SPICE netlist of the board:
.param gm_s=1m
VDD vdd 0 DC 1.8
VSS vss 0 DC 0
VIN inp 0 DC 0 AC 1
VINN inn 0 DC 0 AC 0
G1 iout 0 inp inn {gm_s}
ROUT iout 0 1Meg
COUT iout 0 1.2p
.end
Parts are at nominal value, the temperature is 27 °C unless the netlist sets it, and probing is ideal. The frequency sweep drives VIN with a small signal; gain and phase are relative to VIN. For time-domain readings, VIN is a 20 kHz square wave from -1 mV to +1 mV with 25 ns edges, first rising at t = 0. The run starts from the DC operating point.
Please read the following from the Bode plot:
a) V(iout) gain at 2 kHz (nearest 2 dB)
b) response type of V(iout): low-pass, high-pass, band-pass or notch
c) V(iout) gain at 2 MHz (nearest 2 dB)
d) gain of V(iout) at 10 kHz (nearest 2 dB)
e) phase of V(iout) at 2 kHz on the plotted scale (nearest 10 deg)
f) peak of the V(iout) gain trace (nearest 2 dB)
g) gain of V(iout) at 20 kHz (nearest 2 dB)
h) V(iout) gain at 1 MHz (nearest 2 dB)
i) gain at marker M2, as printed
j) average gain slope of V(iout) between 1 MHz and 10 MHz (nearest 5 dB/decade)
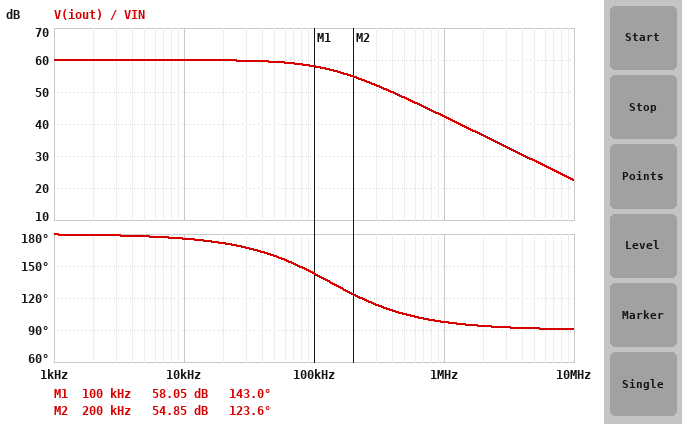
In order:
60 dB
low-pass
36 dB
60 dB
180 deg
60 dB
60 dB
42 dB
54.85 dB
-20 dB/decade
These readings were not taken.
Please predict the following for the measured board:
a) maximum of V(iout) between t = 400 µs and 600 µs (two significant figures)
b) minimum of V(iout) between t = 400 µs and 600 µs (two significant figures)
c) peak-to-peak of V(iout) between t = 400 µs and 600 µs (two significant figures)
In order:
1.0 V
-1.0 V
2.0 V
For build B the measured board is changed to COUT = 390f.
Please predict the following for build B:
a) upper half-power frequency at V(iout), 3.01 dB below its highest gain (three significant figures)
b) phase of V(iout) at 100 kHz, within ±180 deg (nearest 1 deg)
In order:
408 kHz
166 deg
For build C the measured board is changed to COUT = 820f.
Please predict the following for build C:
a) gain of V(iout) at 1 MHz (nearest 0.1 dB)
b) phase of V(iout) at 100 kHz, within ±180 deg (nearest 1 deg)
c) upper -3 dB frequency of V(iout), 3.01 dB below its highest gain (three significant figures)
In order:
45.6 dB
153 deg
194 kHz
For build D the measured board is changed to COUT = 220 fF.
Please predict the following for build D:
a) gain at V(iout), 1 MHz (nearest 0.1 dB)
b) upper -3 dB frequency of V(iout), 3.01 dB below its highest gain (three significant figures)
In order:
55.4 dB
723 kHz
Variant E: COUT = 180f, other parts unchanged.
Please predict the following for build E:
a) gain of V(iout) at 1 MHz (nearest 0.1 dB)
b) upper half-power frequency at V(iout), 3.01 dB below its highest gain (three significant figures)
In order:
56.4 dB
884 kHz
